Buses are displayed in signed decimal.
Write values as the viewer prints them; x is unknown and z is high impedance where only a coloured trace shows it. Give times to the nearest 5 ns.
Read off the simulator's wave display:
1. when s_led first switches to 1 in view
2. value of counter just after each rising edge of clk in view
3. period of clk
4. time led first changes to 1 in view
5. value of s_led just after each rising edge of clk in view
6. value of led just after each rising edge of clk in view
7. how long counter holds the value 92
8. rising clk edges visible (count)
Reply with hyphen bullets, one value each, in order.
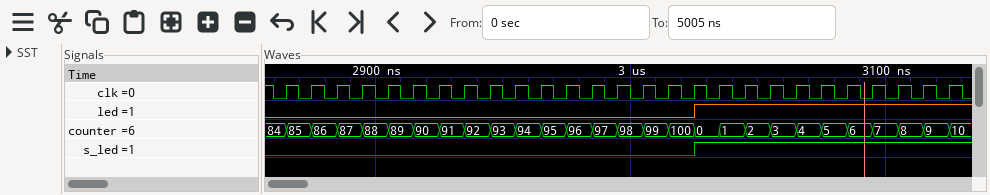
- 3025 ns
- 85, 86, 87, 88, 89, 90, 91, 92, 93, 94, 95, 96, 97, 98, 99, 100, 0, 1, 2, 3, 4, 5, 6, 7, 8, 9, 10
- 10 ns
- 3025 ns
- 0 0 0 0 0 0 0 0 0 0 0 0 0 0 0 0 1 1 1 1 1 1 1 1 1 1 1
- 0 0 0 0 0 0 0 0 0 0 0 0 0 0 0 0 1 1 1 1 1 1 1 1 1 1 1
- 10 ns
- 27
